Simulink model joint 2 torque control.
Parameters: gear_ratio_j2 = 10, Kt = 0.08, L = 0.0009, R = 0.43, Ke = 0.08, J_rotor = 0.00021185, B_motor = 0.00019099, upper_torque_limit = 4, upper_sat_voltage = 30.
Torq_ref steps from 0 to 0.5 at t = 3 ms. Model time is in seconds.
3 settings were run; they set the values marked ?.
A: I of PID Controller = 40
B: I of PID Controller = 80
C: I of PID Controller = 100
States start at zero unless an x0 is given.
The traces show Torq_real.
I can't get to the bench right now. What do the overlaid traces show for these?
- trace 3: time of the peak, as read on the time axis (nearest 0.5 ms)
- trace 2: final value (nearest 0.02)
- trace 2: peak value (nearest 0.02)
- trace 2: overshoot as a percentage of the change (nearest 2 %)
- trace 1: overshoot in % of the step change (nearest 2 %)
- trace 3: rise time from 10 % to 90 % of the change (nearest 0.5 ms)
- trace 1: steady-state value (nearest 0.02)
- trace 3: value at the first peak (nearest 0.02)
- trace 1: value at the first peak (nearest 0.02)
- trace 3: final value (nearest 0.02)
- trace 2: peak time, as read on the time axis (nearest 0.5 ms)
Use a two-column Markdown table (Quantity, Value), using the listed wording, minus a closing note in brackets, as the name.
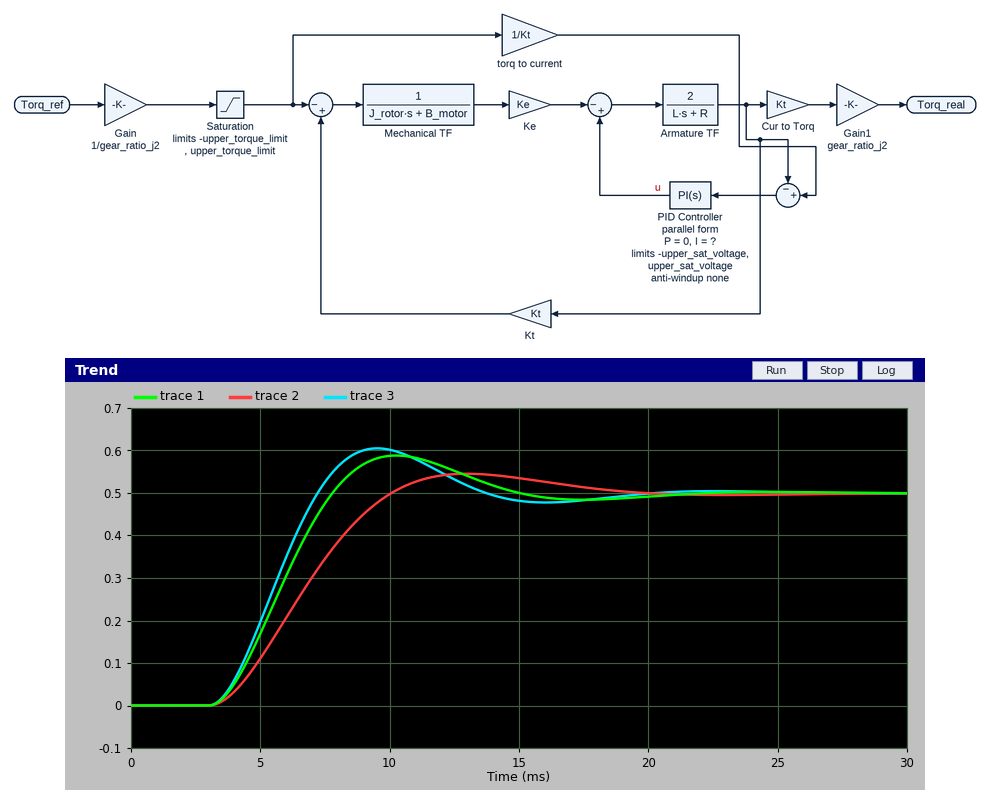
| Quantity | Value |
|---|---|
| trace 3: time of the peak, as read on the time axis | 9.5 ms |
| trace 2: final value | 0.50 |
| trace 2: peak value | 0.54 |
| trace 2: overshoot as a percentage of the change | 10 % |
| trace 1: overshoot in % of the step change | 18 % |
| trace 3: rise time from 10 % to 90 % of the change | 3.0 ms |
| trace 1: steady-state value | 0.50 |
| trace 3: value at the first peak | 0.60 |
| trace 1: value at the first peak | 0.58 |
| trace 3: final value | 0.50 |
| trace 2: peak time, as read on the time axis | 13.0 ms |
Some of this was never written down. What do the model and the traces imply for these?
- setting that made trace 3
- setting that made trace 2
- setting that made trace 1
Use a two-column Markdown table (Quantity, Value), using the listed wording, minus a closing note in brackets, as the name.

| Quantity | Value |
|---|---|
| setting that made trace 3 | C |
| setting that made trace 2 | A |
| setting that made trace 1 | B |
